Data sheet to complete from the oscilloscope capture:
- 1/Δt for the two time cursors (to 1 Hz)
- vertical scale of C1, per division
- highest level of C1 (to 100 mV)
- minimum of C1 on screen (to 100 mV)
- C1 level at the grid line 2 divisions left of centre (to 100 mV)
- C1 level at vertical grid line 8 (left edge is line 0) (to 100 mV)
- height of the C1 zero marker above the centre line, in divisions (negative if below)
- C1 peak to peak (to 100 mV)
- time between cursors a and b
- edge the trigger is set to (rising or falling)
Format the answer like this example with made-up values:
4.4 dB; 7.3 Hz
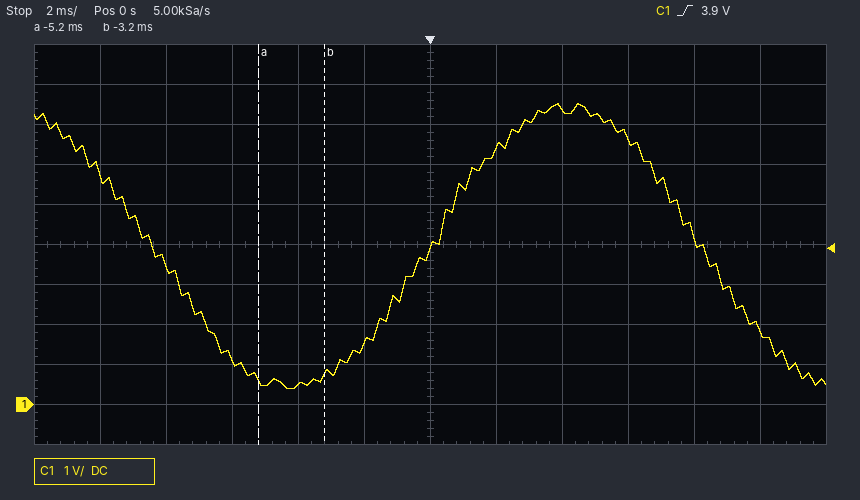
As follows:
500 Hz; 1 V; 7.5 V; 400 mV; 500 mV; 7.4 V; -4.0 div; 7.1 V; 2.0 ms; rising
